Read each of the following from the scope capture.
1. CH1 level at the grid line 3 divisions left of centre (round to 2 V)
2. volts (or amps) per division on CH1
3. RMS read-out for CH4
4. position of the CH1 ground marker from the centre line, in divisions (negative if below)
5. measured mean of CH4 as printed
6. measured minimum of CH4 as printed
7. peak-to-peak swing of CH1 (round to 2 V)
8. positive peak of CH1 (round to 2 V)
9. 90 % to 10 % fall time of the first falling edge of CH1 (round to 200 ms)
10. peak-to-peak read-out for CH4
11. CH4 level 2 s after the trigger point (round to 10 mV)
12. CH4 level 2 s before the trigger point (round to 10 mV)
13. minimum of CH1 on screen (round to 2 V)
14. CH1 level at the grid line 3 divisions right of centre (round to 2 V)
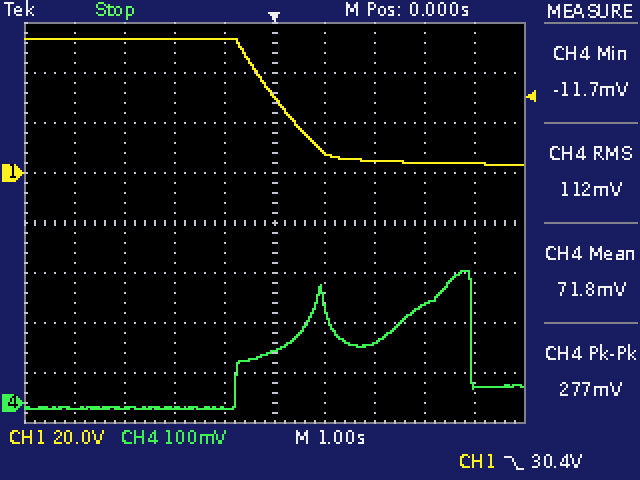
54 V
20 V
112 mV
+1.0 div
71.8 mV
-11.7 mV
50 V
54 V
1.6 s
277 mV
120 mV
-10 mV
4 V
4 V
